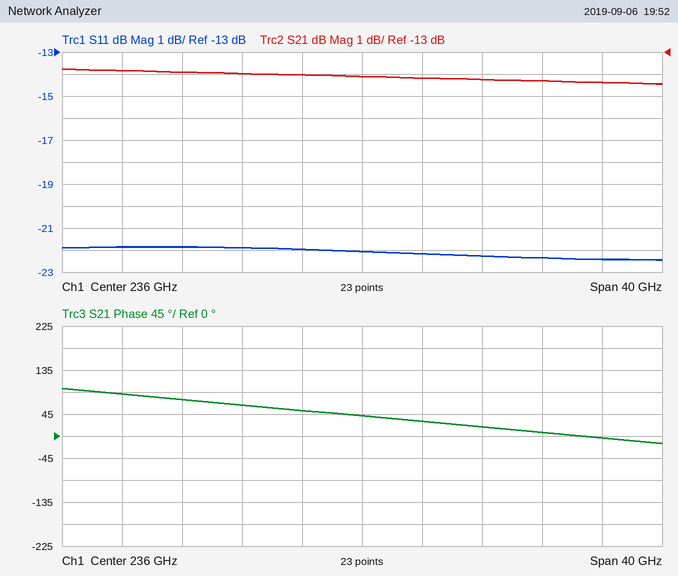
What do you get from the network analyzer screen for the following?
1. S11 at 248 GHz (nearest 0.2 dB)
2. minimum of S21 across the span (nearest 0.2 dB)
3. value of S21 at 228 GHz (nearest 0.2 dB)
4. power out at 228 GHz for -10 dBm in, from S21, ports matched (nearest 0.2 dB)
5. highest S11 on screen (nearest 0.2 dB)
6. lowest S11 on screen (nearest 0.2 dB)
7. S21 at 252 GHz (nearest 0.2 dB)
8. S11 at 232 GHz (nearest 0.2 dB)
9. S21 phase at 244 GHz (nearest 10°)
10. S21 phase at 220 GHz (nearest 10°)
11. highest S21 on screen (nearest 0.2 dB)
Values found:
-22.4 dB
-14.4 dB
-14.0 dB
-24.0 dBm
-21.8 dB
-22.4 dB
-14.4 dB
-22.0 dB
20°
90°
-13.8 dB
